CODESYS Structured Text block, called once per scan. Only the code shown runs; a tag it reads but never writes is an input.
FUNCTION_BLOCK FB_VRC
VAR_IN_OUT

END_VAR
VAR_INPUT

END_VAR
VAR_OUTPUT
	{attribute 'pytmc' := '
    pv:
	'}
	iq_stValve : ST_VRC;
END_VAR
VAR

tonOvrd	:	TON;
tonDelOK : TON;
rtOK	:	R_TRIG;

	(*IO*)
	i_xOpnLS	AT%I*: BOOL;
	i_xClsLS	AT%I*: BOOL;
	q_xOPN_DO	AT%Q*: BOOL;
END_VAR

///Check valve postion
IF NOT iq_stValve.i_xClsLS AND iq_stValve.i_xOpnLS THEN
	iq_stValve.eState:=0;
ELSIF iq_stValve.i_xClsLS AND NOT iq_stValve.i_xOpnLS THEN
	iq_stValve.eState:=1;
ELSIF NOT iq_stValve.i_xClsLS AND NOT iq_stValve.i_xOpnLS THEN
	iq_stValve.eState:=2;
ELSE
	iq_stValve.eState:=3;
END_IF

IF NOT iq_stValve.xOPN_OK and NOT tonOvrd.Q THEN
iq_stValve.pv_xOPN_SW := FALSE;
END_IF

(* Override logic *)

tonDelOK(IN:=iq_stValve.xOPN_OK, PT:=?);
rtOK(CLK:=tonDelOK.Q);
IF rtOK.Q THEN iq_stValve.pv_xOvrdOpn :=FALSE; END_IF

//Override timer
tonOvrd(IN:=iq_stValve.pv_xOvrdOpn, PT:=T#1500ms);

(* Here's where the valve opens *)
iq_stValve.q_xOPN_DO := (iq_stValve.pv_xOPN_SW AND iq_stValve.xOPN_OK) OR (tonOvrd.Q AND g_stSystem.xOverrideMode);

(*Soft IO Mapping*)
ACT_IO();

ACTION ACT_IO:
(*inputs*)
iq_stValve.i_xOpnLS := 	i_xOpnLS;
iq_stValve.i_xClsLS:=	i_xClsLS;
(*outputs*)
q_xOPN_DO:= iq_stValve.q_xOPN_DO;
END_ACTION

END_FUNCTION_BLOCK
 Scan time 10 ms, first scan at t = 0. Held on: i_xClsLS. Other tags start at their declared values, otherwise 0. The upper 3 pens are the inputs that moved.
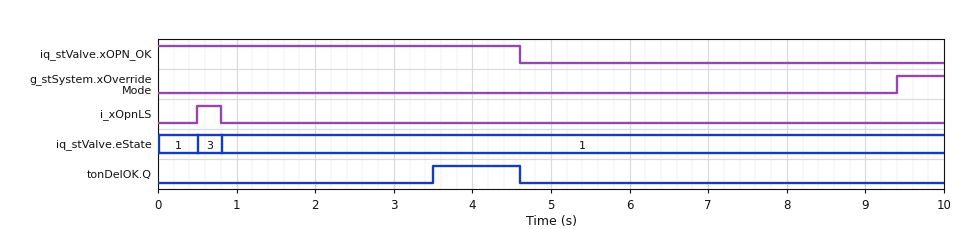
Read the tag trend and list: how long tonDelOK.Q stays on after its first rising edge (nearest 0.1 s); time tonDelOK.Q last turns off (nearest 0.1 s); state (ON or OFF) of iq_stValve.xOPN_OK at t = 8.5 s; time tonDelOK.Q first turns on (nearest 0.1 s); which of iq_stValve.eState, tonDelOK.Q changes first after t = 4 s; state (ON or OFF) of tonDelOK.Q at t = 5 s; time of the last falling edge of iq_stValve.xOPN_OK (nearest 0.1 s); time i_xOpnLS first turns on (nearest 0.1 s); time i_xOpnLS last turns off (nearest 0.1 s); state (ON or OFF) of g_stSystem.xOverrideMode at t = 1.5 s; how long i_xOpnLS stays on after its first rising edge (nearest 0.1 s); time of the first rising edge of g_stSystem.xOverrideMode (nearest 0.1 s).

1.1 s
4.6 s
OFF
3.5 s
tonDelOK.Q
OFF
4.6 s
0.5 s
0.8 s
OFF
0.3 s
9.4 s
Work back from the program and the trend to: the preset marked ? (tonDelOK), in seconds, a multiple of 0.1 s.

3.5 s
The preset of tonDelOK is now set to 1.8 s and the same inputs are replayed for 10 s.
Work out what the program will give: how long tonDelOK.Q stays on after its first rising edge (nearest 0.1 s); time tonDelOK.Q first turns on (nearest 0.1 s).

2.8 s
1.8 s
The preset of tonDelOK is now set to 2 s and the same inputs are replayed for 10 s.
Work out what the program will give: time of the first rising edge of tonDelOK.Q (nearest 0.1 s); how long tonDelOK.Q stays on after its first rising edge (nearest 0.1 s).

2.0 s
2.6 s
